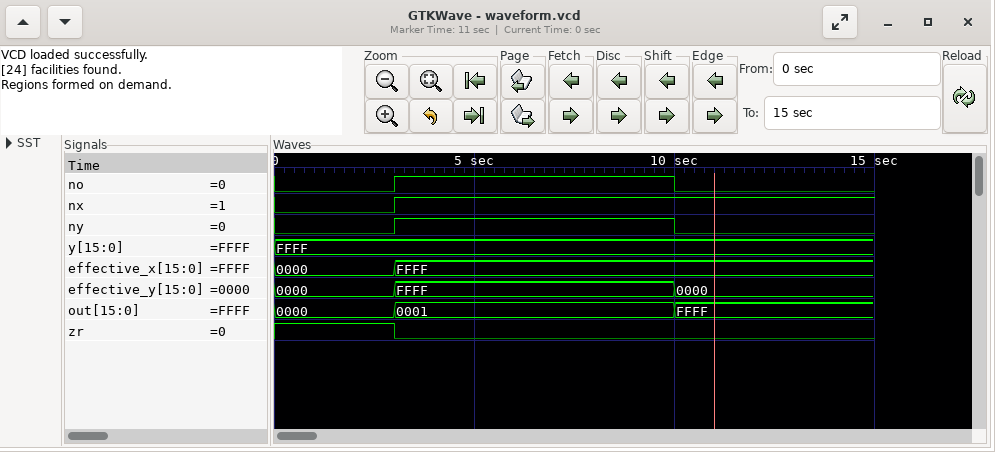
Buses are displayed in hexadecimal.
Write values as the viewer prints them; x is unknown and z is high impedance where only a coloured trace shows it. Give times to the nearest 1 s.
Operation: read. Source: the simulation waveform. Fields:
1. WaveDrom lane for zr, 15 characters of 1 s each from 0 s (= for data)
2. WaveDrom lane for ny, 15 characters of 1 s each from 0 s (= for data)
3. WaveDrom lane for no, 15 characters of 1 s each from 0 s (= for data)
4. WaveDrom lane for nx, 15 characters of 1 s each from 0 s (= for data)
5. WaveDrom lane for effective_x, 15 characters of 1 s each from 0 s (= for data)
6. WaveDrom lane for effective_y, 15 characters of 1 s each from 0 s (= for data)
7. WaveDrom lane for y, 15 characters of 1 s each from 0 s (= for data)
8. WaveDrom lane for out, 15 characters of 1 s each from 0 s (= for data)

{name: 'zr', wave: '1..0...........'}
{name: 'ny', wave: '0..1......0....'}
{name: 'no', wave: '0..1......0....'}
{name: 'nx', wave: '0..1...........'}
{name: 'effective_x', wave: '=..=...........', data: '0000 FFFF'}
{name: 'effective_y', wave: '=..=......=....', data: '0000 FFFF 0000'}
{name: 'y', wave: '=..............', data: 'FFFF'}
{name: 'out', wave: '=..=......=....', data: '0000 0001 FFFF'}
